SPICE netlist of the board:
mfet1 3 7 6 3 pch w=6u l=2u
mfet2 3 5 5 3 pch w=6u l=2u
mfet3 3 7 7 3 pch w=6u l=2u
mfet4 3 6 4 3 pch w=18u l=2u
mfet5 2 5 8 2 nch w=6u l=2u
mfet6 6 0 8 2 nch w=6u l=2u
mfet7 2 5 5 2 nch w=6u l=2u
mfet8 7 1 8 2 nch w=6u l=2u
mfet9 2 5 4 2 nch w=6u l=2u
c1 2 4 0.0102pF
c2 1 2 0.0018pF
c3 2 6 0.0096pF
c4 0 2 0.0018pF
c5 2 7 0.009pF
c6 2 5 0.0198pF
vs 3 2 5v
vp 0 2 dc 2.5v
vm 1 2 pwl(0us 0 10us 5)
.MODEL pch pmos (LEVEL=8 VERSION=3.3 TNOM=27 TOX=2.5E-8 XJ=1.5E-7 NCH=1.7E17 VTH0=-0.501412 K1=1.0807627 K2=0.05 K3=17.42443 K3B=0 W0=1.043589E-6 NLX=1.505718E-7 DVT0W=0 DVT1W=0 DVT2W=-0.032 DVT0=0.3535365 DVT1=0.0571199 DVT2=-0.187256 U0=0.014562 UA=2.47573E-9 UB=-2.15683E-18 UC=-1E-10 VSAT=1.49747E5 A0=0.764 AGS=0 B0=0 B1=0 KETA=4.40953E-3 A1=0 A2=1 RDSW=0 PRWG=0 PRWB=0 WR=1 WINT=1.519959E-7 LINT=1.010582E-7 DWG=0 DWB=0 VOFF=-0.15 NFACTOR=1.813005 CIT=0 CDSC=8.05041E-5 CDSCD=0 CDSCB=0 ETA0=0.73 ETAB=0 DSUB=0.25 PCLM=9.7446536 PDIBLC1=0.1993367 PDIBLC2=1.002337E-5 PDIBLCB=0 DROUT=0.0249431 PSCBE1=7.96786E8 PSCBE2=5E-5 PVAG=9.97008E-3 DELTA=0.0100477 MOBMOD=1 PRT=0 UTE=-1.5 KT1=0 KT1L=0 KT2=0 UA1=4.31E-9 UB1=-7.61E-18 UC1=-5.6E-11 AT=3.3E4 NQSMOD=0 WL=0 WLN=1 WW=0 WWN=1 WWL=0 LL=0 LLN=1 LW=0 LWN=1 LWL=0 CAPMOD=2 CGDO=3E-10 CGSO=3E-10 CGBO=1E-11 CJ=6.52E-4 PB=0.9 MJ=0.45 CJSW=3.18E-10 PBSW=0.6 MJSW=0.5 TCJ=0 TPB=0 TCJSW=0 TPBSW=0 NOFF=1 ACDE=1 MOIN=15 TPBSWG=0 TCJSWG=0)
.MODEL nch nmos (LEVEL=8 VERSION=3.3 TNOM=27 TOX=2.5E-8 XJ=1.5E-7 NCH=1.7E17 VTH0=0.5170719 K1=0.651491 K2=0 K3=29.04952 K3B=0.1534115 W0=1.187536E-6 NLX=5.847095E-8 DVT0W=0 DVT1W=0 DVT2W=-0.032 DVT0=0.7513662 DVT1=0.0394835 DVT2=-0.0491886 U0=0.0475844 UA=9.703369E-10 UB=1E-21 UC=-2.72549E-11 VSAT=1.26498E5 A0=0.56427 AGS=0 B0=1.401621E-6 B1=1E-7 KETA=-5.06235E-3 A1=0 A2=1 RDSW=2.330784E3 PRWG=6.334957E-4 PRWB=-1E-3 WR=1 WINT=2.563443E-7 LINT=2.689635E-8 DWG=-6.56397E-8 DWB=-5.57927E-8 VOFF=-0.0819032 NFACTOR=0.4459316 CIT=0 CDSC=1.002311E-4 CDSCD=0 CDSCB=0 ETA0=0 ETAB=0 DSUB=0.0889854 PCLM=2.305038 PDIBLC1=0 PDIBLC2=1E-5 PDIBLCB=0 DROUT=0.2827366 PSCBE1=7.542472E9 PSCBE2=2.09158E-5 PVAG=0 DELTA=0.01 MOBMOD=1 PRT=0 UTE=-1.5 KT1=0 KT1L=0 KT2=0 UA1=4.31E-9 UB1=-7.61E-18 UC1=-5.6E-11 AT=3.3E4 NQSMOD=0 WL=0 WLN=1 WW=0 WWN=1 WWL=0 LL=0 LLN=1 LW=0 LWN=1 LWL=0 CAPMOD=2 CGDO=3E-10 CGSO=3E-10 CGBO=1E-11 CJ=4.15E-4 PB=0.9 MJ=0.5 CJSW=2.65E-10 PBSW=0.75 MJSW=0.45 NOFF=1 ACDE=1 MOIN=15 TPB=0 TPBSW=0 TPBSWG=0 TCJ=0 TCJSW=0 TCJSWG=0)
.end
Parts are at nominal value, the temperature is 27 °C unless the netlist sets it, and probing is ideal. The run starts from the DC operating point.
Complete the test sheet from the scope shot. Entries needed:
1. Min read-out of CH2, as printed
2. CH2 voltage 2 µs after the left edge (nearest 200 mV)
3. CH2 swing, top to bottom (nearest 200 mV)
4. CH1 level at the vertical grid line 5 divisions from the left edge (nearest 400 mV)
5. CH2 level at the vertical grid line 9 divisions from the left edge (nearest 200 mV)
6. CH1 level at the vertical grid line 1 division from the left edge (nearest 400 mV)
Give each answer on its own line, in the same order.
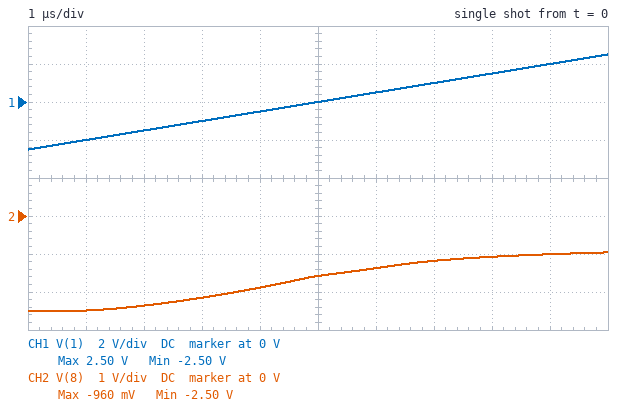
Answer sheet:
-2.50 V
-2.4 V
1.6 V
0 V
-1.0 V
-2.0 V
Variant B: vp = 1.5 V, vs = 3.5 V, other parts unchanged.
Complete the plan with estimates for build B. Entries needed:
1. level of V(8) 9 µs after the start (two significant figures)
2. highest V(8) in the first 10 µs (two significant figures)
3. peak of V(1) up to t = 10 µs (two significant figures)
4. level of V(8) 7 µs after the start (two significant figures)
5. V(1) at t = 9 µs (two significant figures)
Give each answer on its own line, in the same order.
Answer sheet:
-310 mV
-290 mV
3.5 V
-390 mV
3.0 V
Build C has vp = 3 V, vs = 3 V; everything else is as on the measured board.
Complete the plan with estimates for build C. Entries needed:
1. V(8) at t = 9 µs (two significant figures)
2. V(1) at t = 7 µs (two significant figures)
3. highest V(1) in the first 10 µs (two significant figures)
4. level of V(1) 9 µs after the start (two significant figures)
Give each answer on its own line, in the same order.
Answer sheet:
-1.5 V
500 mV
2.0 V
1.5 V
